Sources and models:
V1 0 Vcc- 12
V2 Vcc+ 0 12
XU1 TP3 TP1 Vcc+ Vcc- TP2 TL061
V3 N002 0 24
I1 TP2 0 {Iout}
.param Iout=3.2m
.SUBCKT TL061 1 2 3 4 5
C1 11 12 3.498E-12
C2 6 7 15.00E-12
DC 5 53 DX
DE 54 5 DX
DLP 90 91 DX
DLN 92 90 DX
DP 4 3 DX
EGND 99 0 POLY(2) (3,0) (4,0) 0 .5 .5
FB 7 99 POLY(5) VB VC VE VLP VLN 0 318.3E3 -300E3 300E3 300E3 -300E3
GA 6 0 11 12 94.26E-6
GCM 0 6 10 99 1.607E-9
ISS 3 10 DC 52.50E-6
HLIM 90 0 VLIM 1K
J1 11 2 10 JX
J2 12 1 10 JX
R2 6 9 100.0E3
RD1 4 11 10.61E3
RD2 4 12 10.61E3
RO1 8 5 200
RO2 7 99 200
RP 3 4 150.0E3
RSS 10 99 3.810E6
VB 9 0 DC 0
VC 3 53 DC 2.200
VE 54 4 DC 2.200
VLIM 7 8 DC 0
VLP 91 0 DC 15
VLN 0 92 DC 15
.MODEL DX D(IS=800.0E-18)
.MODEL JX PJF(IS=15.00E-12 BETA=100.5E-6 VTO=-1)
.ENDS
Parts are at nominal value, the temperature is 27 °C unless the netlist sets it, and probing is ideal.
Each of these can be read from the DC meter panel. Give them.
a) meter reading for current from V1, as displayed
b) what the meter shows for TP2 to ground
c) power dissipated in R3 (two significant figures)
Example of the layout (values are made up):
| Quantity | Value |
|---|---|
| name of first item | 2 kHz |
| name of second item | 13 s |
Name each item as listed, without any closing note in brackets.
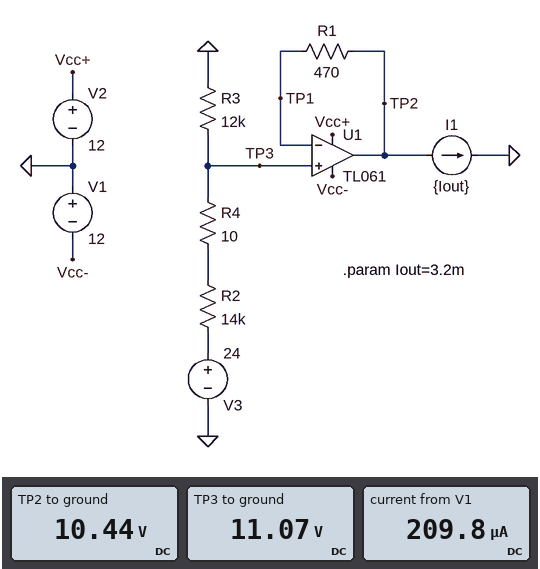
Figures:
| Quantity | Value |
|---|---|
| meter reading for current from V1, as displayed | 209.8 µA |
| what the meter shows for TP2 to ground | 10.44 V |
| power dissipated in R3 | 10 mW |
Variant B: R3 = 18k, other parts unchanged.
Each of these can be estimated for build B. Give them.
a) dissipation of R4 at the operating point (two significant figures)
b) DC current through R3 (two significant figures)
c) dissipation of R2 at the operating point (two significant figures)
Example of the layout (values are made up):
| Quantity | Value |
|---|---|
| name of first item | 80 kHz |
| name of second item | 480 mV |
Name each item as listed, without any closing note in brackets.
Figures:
| Quantity | Value |
|---|---|
| dissipation of R4 at the operating point | 5.6 µW |
| DC current through R3 | 750 µA |
| dissipation of R2 at the operating point | 7.9 mW |
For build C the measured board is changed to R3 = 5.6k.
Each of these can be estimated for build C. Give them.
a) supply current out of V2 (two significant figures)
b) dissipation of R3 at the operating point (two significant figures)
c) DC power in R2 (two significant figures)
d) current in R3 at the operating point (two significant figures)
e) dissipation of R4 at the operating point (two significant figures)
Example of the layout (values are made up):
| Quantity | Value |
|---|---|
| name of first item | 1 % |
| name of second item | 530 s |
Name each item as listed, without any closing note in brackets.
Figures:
| Quantity | Value |
|---|---|
| supply current out of V2 | 210 µA |
| dissipation of R3 at the operating point | 8.4 mW |
| DC power in R2 | 21 mW |
| current in R3 at the operating point | 1.2 mA |
| dissipation of R4 at the operating point | 15 µW |
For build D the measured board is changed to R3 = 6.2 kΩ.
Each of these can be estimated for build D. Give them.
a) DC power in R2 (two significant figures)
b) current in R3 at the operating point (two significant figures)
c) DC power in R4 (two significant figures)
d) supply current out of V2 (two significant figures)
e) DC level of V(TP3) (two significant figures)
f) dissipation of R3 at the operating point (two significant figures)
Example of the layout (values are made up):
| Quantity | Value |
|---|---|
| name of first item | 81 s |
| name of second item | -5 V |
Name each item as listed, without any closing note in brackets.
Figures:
| Quantity | Value |
|---|---|
| DC power in R2 | 20 mW |
| current in R3 at the operating point | 1.2 mA |
| DC power in R4 | 14 µW |
| supply current out of V2 | 210 µA |
| DC level of V(TP3) | 7.4 V |
| dissipation of R3 at the operating point | 8.7 mW |
